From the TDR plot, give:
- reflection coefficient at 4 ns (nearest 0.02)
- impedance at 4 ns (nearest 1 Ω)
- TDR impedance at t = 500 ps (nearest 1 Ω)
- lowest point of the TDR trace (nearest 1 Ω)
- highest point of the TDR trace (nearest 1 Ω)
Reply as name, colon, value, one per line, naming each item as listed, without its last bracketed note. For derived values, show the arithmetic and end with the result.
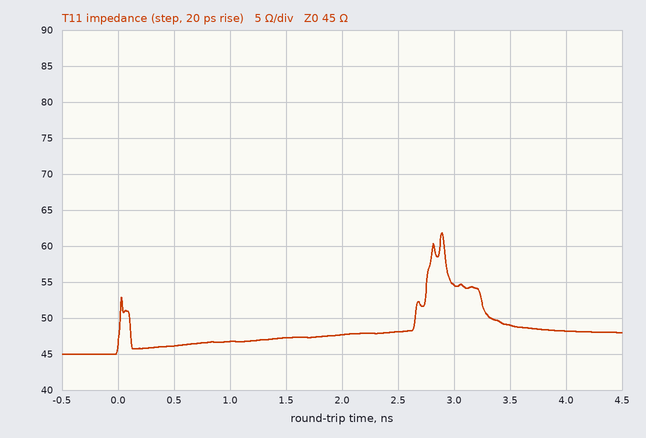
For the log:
reflection coefficient at 4 ns: (48 − 45)/(48 + 45) ≈ +0.0323, so +0.04 to the nearest 0.02
impedance at 4 ns: 48 Ω
TDR impedance at t = 500 ps: 46 Ω
lowest point of the TDR trace: 45 Ω
highest point of the TDR trace: 62 Ω
